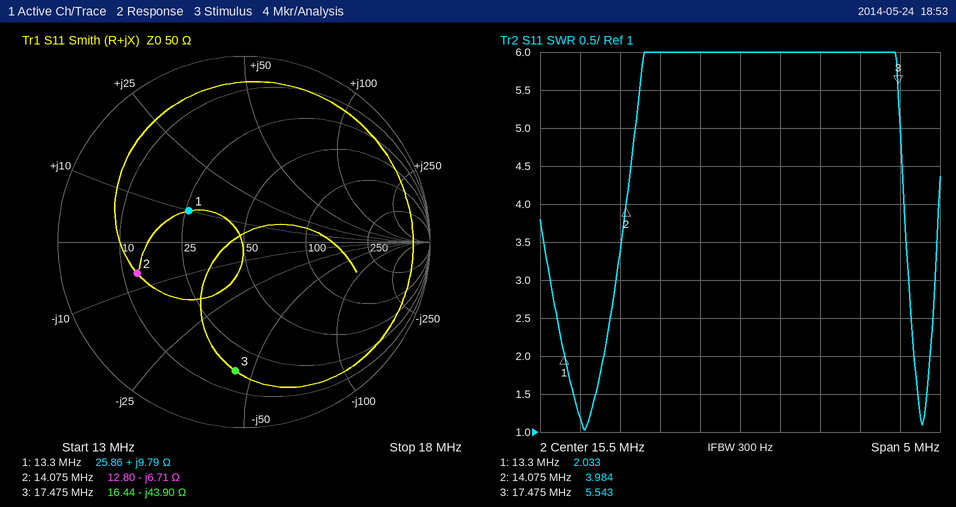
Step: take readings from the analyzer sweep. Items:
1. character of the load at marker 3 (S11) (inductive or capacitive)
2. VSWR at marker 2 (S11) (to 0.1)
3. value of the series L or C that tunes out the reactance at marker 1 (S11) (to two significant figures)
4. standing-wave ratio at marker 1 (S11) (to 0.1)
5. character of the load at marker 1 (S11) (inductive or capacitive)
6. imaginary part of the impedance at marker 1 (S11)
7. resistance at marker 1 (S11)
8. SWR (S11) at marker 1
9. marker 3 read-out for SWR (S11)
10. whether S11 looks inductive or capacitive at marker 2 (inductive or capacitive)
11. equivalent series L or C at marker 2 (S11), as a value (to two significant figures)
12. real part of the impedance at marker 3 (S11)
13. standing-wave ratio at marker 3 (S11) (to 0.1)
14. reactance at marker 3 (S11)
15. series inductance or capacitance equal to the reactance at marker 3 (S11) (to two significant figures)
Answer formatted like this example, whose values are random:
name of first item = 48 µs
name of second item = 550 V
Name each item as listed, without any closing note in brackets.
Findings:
character of the load at marker 3 (S11) = capacitive
VSWR at marker 2 (S11) = 4.0
value of the series L or C that tunes out the reactance at marker 1 (S11) = 1.2 nF
standing-wave ratio at marker 1 (S11) = 2.0
character of the load at marker 1 (S11) = inductive
imaginary part of the impedance at marker 1 = +9.79 Ω
resistance at marker 1 = 25.86 Ω
SWR (S11) at marker 1 = 2.033
marker 3 read-out for SWR = 5.543
whether S11 looks inductive or capacitive at marker 2 = capacitive
equivalent series L or C at marker 2 (S11), as a value = 1.7 nF
real part of the impedance at marker 3 = 16.44 Ω
standing-wave ratio at marker 3 (S11) = 5.5
reactance at marker 3 = -43.90 Ω
series inductance or capacitance equal to the reactance at marker 3 (S11) = 210 pF
